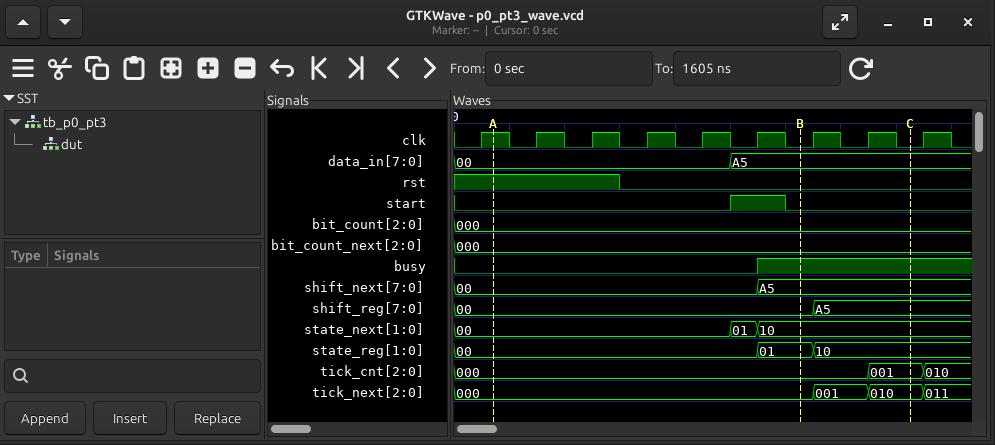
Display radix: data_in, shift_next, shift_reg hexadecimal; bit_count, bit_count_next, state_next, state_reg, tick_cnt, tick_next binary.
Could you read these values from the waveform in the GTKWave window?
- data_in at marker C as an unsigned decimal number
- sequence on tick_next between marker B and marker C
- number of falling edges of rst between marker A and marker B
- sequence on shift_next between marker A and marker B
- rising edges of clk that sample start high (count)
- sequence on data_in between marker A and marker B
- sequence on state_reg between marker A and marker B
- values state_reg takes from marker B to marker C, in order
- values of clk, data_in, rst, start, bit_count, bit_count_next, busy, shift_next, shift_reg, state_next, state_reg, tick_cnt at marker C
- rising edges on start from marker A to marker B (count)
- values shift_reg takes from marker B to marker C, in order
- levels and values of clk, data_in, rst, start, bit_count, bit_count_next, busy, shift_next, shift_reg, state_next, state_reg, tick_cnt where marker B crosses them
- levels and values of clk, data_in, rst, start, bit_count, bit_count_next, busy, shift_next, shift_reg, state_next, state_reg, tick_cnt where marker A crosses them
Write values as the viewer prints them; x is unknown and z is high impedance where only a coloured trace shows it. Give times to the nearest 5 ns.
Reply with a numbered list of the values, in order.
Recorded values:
1. 165
2. 000, 001, 010
3. 1
4. 00, A5
5. 1
6. 00, A5
7. 00, 01
8. 01, 10
9. clk=0, data_in=A5, rst=0, start=0, bit_count=000, bit_count_next=000, busy=1, shift_next=A5, shift_reg=A5, state_next=10, state_reg=10, tick_cnt=001
10. 1
11. 00, A5
12. clk=0, data_in=A5, rst=0, start=0, bit_count=000, bit_count_next=000, busy=1, shift_next=A5, shift_reg=00, state_next=10, state_reg=01, tick_cnt=000
13. clk=1, data_in=00, rst=1, start=0, bit_count=000, bit_count_next=000, busy=0, shift_next=00, shift_reg=00, state_next=00, state_reg=00, tick_cnt=000
